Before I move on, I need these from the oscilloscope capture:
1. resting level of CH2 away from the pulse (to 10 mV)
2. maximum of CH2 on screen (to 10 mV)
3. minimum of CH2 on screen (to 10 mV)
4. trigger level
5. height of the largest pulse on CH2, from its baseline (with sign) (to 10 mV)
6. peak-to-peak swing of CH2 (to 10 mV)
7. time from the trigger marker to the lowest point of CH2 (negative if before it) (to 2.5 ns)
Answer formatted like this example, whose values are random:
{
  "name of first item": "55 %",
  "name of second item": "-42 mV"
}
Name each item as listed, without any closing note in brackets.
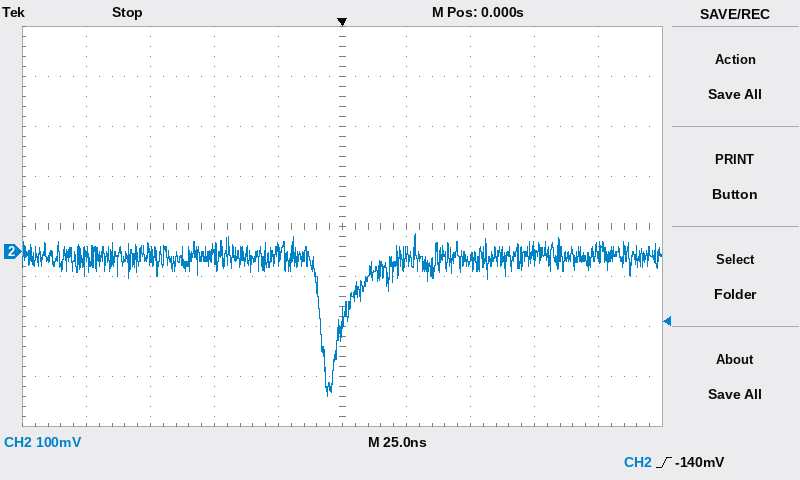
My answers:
{
  "resting level of CH2 away from the pulse": "-10 mV",
  "maximum of CH2 on screen": "40 mV",
  "minimum of CH2 on screen": "-290 mV",
  "trigger level": "-140 mV",
  "height of the largest pulse on CH2, from its baseline (with sign)": "-280 mV",
  "peak-to-peak swing of CH2": "330 mV",
  "time from the trigger marker to the lowest point of CH2 (negative if before it)": "-5.0 ns"
}
